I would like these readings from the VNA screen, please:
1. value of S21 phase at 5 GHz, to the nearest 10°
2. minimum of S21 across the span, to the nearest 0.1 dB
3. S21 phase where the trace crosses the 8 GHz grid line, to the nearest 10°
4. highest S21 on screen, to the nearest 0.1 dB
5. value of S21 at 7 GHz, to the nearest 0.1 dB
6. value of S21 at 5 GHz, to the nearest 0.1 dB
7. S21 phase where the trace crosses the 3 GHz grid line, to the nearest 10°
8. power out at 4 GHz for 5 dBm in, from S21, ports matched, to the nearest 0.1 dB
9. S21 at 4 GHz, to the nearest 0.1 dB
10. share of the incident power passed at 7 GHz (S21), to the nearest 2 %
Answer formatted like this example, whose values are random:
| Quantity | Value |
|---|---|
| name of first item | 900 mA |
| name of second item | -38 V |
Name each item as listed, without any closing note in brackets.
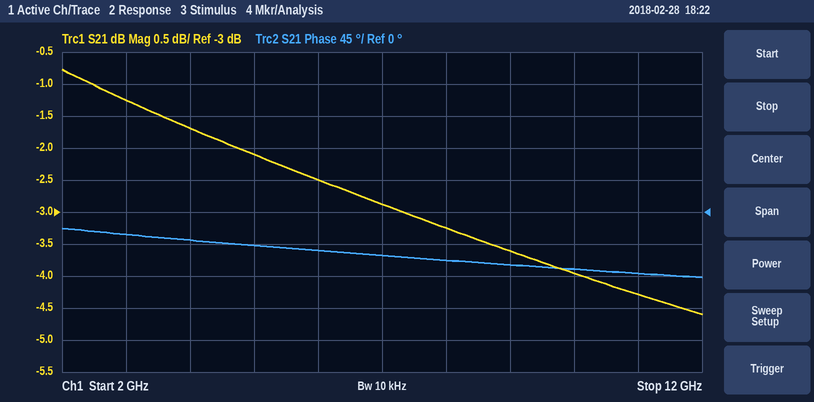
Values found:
| Quantity | Value |
|---|---|
| value of S21 phase at 5 GHz, to the nearest 10° | -50° |
| minimum of S21 across the span, to the nearest 0.1 dB | -4.6 dB |
| S21 phase where the trace crosses the 8 GHz grid line, to the nearest 10° | -70° |
| highest S21 on screen, to the nearest 0.1 dB | -0.8 dB |
| value of S21 at 7 GHz, to the nearest 0.1 dB | -2.9 dB |
| value of S21 at 5 GHz, to the nearest 0.1 dB | -2.1 dB |
| S21 phase where the trace crosses the 3 GHz grid line, to the nearest 10° | -30° |
| power out at 4 GHz for 5 dBm in, from S21, ports matched, to the nearest 0.1 dB | 3.3 dBm |
| S21 at 4 GHz, to the nearest 0.1 dB | -1.7 dB |
| share of the incident power passed at 7 GHz (S21), to the nearest 2 % | 52 % |
